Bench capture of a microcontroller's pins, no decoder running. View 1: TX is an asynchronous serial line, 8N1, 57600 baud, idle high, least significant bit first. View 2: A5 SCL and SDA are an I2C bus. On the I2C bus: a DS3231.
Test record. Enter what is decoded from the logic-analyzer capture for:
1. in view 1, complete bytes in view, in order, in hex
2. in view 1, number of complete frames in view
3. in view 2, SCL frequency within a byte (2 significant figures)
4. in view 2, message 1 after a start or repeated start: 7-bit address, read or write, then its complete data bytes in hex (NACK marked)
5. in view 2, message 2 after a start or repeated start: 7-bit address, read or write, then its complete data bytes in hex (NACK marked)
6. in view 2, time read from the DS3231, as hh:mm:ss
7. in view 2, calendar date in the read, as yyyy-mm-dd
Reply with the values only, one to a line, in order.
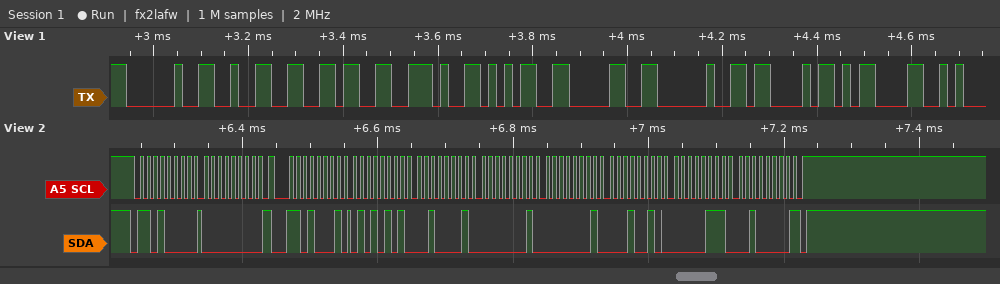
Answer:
20 32 36 2E 35 30 20 43 0D
9
100 kHz
0x68 write: 00
0x68 read: 55 21 01 01 12 07 20 NACK
01:21:55
2020-07-12
